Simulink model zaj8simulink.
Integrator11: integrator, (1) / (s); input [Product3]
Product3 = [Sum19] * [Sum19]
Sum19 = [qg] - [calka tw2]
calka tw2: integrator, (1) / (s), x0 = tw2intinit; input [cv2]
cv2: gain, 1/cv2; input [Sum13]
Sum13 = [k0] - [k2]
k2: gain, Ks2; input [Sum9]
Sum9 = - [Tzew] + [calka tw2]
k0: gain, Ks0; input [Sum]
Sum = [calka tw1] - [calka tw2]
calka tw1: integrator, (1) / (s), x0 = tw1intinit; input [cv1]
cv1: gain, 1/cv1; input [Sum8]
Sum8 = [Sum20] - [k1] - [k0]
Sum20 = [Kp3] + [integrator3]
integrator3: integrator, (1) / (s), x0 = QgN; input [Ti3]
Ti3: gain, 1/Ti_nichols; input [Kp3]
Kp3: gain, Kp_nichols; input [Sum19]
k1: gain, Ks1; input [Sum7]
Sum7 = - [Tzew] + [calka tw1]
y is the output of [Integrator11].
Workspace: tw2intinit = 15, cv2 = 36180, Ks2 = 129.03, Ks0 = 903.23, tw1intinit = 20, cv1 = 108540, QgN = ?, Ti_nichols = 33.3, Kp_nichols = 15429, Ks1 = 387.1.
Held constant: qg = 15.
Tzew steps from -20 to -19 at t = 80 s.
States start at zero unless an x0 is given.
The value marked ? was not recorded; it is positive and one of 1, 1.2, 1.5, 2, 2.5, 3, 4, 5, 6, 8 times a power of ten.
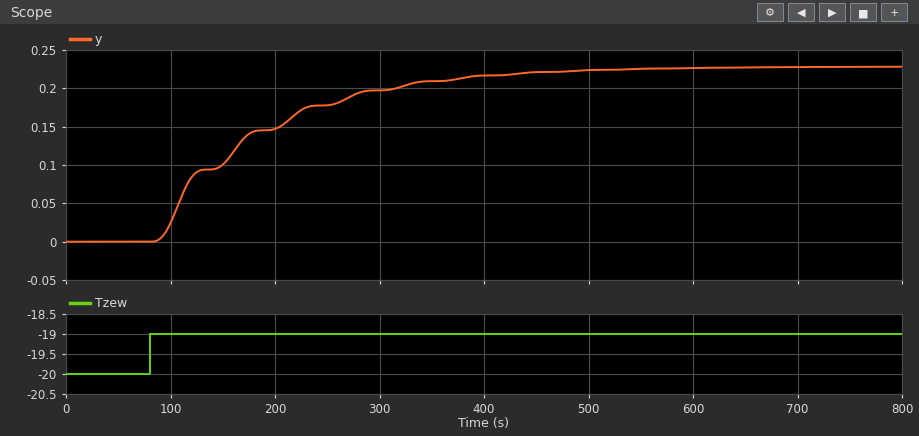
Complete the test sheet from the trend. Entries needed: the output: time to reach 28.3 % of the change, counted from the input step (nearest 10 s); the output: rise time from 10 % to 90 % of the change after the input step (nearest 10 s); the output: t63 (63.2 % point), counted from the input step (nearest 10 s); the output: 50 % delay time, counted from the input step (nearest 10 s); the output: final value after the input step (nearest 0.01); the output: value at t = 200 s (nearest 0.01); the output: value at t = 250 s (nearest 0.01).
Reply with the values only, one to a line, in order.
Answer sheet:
30 s
230 s
100 s
80 s
0.23
0.15
0.18
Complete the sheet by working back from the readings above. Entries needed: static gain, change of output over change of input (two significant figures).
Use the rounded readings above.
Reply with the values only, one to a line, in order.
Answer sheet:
0.23
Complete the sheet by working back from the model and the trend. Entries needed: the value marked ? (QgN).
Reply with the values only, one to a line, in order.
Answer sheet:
20000
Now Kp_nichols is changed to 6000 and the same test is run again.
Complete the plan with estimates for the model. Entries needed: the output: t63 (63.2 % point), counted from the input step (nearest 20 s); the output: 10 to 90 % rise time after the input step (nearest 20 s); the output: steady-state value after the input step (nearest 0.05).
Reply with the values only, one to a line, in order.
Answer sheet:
140 s
280 s
0.75
